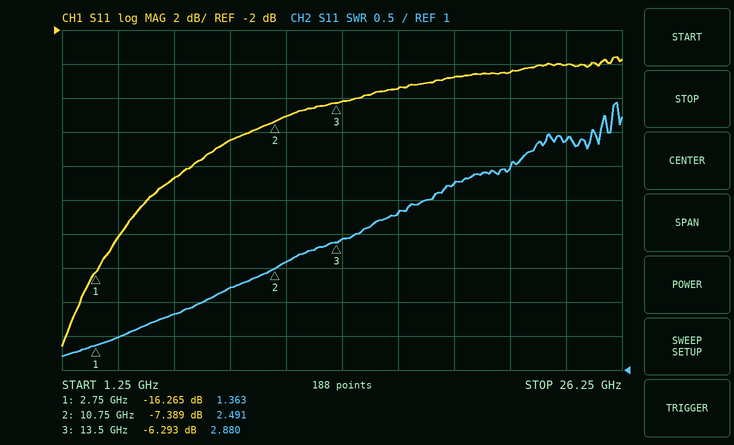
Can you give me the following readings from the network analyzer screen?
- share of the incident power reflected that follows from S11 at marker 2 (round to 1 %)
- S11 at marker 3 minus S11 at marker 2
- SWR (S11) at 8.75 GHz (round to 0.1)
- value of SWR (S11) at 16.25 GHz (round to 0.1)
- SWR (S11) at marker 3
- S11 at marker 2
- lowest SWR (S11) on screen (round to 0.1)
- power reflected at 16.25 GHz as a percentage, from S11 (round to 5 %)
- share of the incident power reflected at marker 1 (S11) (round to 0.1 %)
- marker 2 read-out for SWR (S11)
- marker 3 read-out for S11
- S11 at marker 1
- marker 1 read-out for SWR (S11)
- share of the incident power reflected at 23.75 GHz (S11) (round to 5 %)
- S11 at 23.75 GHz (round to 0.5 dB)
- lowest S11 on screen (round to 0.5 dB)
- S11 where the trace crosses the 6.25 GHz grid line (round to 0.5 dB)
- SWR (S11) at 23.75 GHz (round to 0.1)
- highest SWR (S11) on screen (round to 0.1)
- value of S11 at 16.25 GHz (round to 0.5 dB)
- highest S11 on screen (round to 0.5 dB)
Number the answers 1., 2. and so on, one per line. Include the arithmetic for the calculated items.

1. 10^(-7.389/10) ≈ 18 %
2. -6.293 − (-7.389) = 1.096 dB
3. 2.2
4. 3.3
5. 2.880
6. -7.389 dB
7. 1.2
8. 10^(-5.5/10) ≈ 28.2 %, so 30 % to the nearest 5 %
9. 10^(-16.265/10) ≈ 2.4 %
10. 2.491
11. -6.293 dB
12. -16.265 dB
13. 1.363
14. 10^(-4/10) ≈ 40 %
15. -4.0 dB
16. -20.5 dB
17. -10.5 dB
18. 4.4
19. 4.9
20. -5.5 dB
21. -3.5 dB
